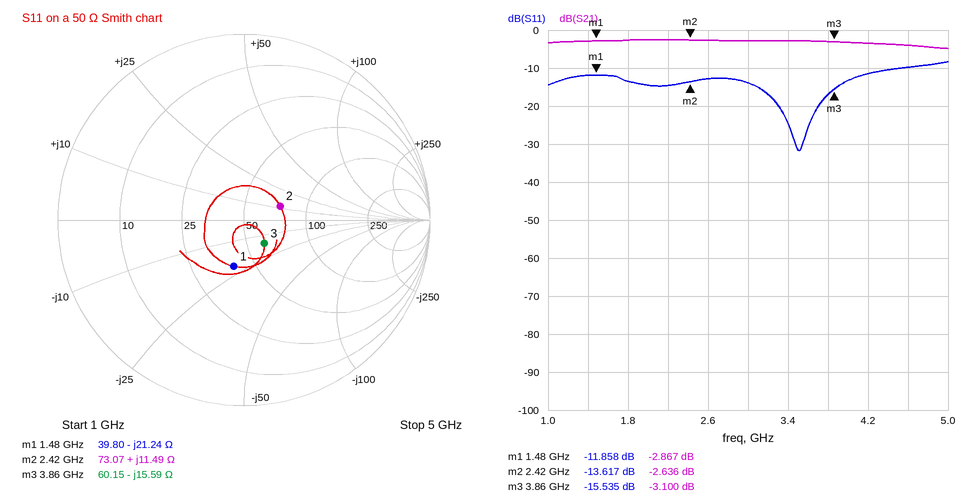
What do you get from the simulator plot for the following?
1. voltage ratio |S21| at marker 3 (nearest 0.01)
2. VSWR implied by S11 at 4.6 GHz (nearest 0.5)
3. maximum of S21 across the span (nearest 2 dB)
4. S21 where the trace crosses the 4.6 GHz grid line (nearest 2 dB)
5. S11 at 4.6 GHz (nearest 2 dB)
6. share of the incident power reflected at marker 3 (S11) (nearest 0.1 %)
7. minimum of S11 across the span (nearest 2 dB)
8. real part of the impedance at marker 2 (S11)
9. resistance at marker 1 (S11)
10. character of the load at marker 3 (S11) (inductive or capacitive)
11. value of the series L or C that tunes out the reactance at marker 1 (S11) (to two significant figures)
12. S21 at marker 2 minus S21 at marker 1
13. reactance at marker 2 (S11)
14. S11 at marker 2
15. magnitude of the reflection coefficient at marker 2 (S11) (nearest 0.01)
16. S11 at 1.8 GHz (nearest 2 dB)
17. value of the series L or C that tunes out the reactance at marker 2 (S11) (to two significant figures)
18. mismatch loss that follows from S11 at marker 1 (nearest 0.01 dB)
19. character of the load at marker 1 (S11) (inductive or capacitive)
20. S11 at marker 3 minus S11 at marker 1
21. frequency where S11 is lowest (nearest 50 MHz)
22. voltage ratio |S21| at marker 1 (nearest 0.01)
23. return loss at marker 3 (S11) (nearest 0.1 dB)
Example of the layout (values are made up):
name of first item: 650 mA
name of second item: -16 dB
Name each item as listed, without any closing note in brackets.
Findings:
voltage ratio |S21| at marker 3: 0.70
VSWR implied by S11 at 4.6 GHz: 2.0
maximum of S21 across the span: -2 dB
S21 where the trace crosses the 4.6 GHz grid line: -4 dB
S11 at 4.6 GHz: -10 dB
share of the incident power reflected at marker 3 (S11): 2.8 %
minimum of S11 across the span: -32 dB
real part of the impedance at marker 2: 73.07 Ω
resistance at marker 1: 39.80 Ω
character of the load at marker 3 (S11): capacitive
value of the series L or C that tunes out the reactance at marker 1 (S11): 2.3 nH
S21 at marker 2 minus S21 at marker 1: 0.231 dB
reactance at marker 2: +11.49 Ω
S11 at marker 2: -13.617 dB
magnitude of the reflection coefficient at marker 2 (S11): 0.21
S11 at 1.8 GHz: -14 dB
value of the series L or C that tunes out the reactance at marker 2 (S11): 5.7 pF
mismatch loss that follows from S11 at marker 1: 0.29 dB
character of the load at marker 1 (S11): capacitive
S11 at marker 3 minus S11 at marker 1: -3.677 dB
frequency where S11 is lowest: 3.50 GHz
voltage ratio |S21| at marker 1: 0.72
return loss at marker 3 (S11): 15.5 dB
